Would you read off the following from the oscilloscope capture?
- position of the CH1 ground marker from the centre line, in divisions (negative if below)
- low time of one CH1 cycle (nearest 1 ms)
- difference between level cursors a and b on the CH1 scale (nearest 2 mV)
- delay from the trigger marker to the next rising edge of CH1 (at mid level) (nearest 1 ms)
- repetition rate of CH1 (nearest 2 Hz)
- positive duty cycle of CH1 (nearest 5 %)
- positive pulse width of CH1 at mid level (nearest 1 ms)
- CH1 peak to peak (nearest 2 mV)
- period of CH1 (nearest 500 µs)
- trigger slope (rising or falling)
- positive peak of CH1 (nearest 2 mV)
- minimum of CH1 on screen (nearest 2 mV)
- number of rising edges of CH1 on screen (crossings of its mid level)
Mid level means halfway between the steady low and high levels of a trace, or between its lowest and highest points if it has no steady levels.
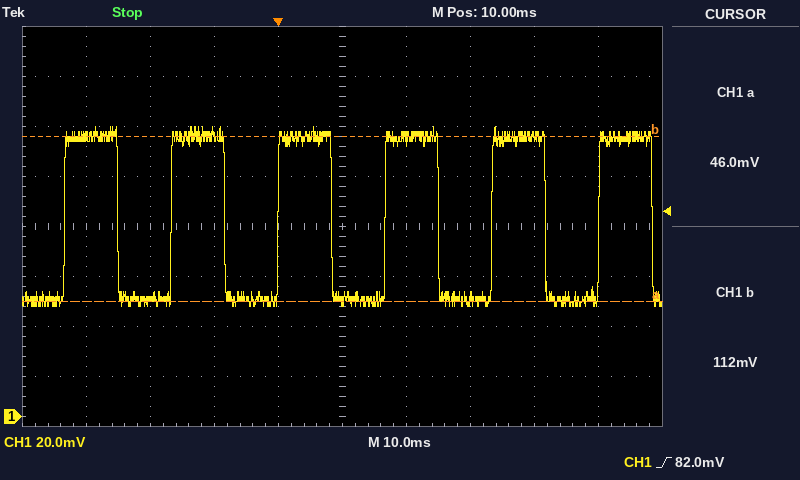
-3.8 div
8 ms
66 mV
17 ms
60 Hz
50 %
8 ms
72 mV
16.5 ms
rising
116 mV
44 mV
6
